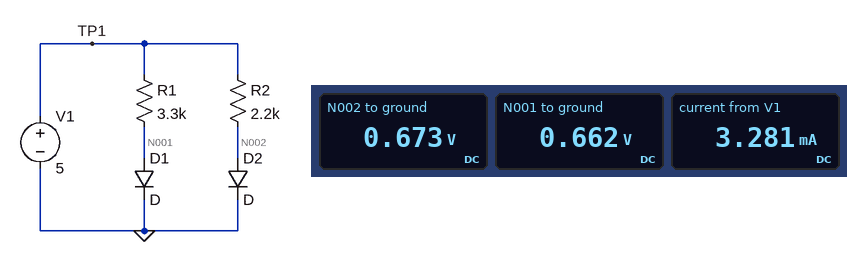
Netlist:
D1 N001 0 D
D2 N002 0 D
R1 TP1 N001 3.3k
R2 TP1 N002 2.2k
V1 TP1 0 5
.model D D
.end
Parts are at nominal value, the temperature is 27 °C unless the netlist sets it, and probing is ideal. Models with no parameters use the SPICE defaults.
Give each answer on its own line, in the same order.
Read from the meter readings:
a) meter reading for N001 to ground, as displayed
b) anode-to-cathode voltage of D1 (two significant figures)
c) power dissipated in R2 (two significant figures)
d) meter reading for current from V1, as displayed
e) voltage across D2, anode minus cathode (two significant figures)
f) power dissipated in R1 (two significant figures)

0.662 V
660 mV
8.5 mW
3.281 mA
670 mV
5.7 mW
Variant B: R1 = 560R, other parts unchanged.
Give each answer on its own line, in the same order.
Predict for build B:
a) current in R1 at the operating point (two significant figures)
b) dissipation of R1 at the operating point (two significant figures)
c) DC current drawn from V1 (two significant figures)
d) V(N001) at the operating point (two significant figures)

7.7 mA
33 mW
9.6 mA
710 mV
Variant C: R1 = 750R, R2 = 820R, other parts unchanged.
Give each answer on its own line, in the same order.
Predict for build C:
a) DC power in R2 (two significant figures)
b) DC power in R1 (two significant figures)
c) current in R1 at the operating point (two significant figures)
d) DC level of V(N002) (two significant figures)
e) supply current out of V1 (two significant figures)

23 mW
25 mW
5.7 mA
700 mV
11 mA
